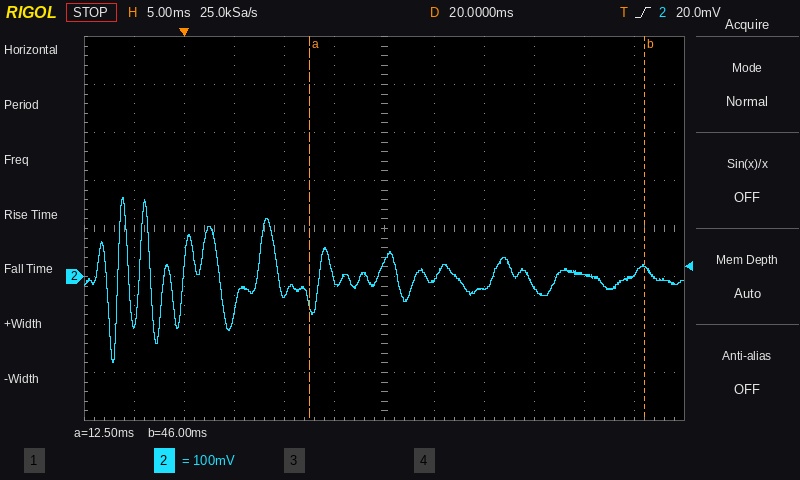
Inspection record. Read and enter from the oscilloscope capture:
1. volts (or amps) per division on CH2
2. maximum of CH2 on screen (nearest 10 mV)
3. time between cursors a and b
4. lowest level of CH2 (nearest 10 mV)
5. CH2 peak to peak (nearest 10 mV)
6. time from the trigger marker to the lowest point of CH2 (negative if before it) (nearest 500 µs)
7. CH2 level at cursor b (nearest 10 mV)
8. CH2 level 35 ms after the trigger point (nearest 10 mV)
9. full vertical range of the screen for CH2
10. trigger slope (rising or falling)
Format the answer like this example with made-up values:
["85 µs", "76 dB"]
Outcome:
["100 mV", "160 mV", "33.5 ms", "-180 mV", "340 mV", "-7.0 ms", "20 mV", "-20 mV", "800 mV", "rising"]
